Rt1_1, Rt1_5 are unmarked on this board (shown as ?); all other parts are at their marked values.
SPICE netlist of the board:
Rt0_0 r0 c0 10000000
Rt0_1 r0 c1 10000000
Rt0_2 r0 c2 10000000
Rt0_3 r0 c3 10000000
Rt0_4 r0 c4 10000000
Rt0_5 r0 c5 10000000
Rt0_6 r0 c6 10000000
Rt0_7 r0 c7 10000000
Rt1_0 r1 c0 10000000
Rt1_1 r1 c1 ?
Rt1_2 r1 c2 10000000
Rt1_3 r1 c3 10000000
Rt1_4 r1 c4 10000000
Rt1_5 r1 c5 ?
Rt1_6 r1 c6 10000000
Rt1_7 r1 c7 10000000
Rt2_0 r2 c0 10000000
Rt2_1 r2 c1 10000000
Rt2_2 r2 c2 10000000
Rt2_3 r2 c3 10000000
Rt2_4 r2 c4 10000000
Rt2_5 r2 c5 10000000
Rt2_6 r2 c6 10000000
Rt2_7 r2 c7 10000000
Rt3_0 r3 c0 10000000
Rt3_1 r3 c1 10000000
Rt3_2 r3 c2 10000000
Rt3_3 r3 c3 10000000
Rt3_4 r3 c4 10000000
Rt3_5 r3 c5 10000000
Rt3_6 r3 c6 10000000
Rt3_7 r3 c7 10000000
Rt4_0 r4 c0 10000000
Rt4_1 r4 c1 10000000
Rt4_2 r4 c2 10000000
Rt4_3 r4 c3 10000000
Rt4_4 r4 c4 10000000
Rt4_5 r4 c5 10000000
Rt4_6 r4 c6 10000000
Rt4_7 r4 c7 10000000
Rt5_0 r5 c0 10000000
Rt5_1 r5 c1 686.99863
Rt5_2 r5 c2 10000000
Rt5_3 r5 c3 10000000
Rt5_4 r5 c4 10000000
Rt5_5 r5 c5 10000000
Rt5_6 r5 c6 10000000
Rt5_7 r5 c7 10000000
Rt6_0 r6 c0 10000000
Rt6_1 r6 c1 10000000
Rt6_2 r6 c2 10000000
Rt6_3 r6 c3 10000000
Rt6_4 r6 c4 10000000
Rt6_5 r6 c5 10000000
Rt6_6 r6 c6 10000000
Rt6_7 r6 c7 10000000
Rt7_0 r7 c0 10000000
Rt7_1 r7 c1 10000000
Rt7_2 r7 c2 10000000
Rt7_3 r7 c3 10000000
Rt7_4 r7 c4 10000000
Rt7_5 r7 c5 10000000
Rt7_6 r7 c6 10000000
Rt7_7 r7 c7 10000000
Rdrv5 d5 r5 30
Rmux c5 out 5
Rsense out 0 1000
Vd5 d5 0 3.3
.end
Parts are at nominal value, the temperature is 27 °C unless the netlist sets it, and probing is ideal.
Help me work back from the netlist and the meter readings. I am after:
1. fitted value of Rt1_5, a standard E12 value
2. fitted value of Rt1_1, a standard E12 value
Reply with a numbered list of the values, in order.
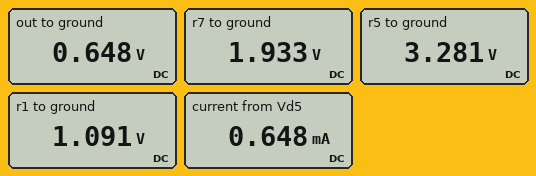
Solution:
1. 680 Ω
2. 2.7 kΩ
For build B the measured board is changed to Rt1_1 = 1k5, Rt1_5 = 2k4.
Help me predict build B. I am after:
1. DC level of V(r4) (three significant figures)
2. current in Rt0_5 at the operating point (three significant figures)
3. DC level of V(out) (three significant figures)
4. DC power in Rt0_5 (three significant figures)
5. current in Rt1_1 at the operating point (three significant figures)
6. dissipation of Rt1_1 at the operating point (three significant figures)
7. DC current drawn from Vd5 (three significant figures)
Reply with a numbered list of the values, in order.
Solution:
1. 2.12 V
2. 153 nA
3. 588 mV
4. 235 nW
5. 587 µA
6. 516 µW
7. 588 µA
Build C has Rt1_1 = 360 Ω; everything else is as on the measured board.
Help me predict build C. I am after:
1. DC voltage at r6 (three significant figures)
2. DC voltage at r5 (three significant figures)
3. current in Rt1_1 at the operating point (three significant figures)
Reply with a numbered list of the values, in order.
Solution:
1. 2.17 V
2. 3.26 V
3. 1.19 mA
